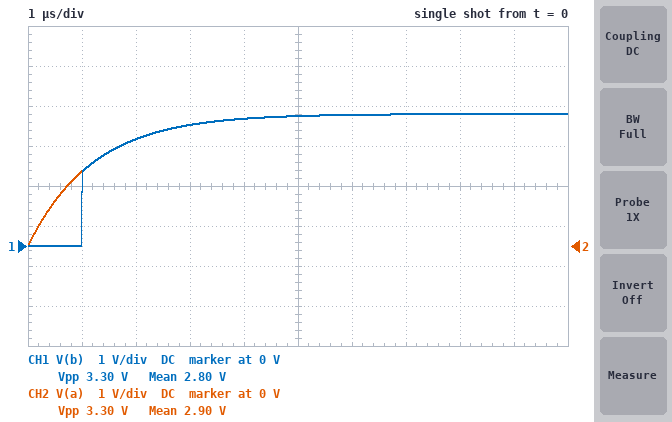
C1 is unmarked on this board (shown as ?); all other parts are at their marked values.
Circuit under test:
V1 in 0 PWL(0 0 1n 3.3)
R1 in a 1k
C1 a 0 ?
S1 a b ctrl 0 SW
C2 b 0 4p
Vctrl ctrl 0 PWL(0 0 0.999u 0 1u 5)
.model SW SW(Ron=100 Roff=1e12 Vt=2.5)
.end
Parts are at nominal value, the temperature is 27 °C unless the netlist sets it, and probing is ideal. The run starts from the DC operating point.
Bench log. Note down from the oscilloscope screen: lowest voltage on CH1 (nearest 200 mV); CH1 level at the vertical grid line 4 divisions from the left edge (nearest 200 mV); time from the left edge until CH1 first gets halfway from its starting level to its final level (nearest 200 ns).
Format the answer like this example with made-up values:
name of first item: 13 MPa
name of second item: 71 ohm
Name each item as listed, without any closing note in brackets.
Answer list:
lowest voltage on CH1: 0 V
CH1 level at the vertical grid line 4 divisions from the left edge: 3.2 V
time from the left edge until CH1 first gets halfway from its starting level to its final level: 1.0 µs
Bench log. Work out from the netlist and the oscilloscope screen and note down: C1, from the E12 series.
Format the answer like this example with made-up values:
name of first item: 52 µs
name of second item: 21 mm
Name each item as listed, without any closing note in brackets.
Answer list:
C1, from the E12 series: 1.2 nF
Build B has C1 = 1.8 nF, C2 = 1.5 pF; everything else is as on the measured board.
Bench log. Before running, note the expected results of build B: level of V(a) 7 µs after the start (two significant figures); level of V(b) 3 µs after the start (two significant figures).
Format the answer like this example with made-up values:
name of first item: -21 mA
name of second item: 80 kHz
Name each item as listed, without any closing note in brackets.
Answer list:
level of V(a) 7 µs after the start: 3.2 V
level of V(b) 3 µs after the start: 2.7 V
